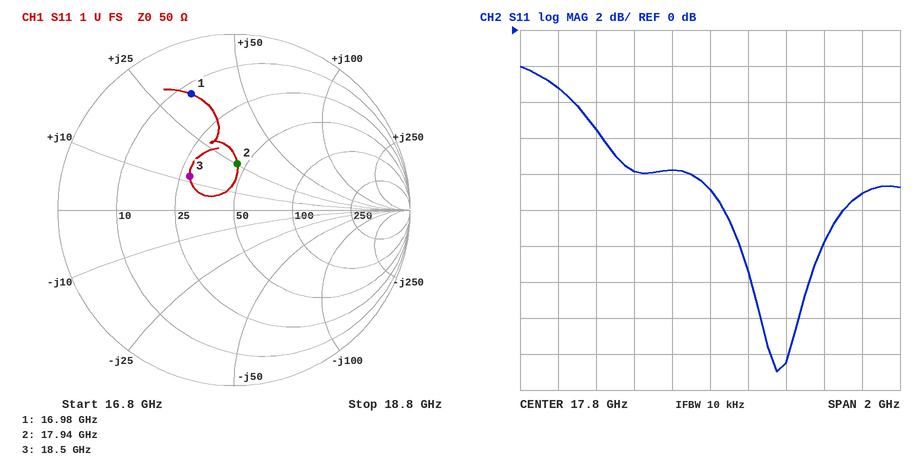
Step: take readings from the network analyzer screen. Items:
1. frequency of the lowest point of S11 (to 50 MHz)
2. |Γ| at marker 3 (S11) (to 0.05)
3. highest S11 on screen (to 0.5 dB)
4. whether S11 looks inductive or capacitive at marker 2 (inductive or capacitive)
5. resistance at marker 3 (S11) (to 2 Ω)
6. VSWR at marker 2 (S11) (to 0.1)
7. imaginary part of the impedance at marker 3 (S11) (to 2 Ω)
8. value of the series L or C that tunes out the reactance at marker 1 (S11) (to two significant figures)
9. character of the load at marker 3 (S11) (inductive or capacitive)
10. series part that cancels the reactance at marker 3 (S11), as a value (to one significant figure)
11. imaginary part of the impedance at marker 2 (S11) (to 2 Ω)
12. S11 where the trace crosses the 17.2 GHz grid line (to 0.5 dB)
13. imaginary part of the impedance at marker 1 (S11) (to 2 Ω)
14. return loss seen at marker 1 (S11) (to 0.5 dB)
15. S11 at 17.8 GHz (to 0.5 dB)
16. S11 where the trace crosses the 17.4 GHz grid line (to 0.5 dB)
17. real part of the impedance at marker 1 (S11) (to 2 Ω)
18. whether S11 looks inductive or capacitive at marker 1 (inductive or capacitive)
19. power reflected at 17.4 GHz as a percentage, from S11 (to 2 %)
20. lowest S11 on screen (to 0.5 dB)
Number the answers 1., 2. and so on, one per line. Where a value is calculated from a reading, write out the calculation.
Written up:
1. 18.15 GHz
2. 0.30
3. -2.0 dB
4. inductive
5. 28 Ω
6. 1.7
7. +12 Ω
8. C = 1/(2π × 16.98 GHz × 34 Ω) ≈ 276 fF, so 280 fF to two significant figures
9. inductive
10. C = 1/(2π × 18.5 GHz × 12 Ω) ≈ 717 fF, so 700 fF to one significant figure
11. +26 Ω
12. -5.5 dB
13. +34 Ω
14. 3.0 dB
15. -9.0 dB
16. -8.0 dB
17. 12 Ω
18. inductive
19. 10^(-8/10) ≈ 16 %
20. -19.0 dB
